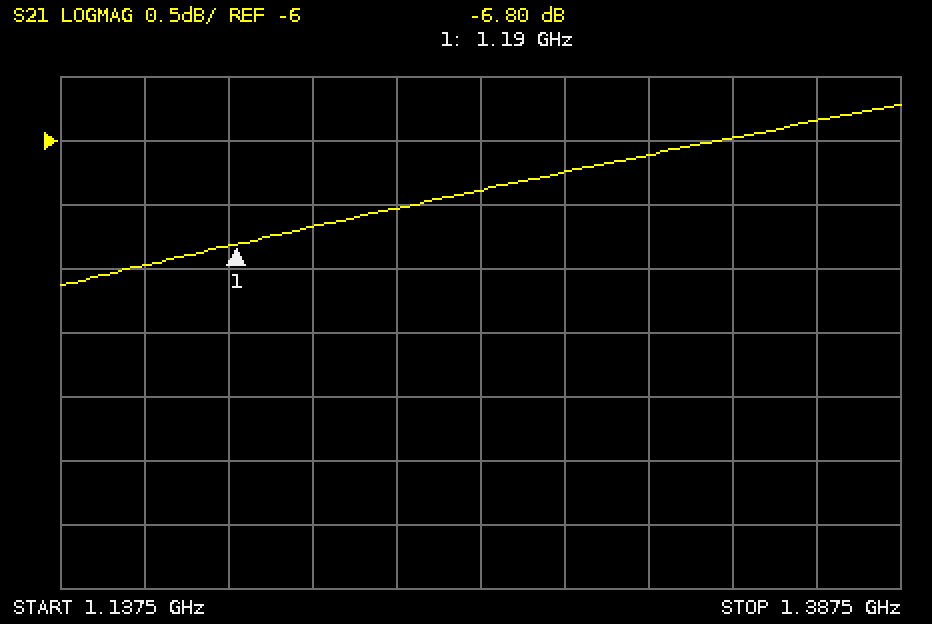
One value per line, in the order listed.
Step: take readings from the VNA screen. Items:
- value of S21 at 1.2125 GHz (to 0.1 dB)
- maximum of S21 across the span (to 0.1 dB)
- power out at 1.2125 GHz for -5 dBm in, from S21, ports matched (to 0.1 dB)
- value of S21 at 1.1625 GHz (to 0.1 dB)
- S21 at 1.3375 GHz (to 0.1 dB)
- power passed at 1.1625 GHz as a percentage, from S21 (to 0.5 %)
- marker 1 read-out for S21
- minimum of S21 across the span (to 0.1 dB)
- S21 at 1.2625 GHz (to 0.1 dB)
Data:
-6.7 dB
-5.7 dB
-11.7 dBm
-7.0 dB
-6.0 dB
20.0 %
-6.80 dB
-7.1 dB
-6.4 dB
